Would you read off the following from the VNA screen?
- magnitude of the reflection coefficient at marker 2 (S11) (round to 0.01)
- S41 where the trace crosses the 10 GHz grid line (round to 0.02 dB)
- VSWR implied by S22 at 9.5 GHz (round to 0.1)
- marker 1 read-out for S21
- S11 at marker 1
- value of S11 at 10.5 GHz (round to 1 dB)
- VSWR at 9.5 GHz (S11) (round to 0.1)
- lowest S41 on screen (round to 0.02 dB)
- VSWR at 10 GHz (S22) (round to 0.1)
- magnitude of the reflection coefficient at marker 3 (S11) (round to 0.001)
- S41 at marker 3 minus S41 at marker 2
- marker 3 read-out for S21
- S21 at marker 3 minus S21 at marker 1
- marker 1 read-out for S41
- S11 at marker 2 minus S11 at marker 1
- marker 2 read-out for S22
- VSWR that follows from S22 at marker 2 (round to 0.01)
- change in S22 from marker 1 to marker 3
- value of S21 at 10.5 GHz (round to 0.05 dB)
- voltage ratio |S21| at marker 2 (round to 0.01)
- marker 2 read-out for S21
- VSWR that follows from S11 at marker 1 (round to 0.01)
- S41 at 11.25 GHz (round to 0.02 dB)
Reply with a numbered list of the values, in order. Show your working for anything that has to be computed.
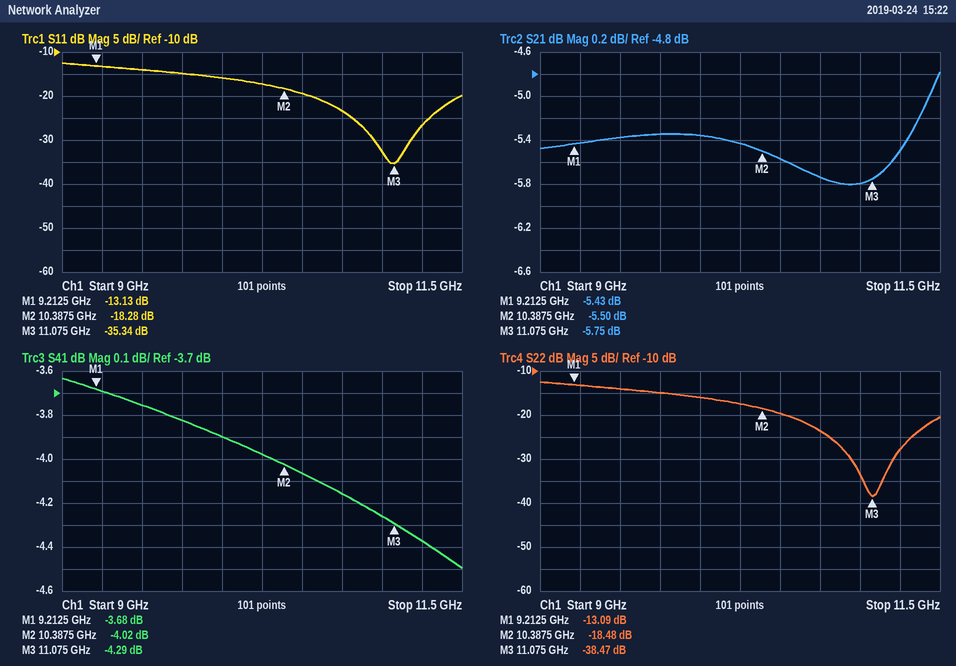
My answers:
1. 10^(-18.28/20) ≈ 0.12
2. -3.90 dB
3. |Γ| = 10^(-14/20) = 0.1995; VSWR = (1 + 0.1995)/(1 − 0.1995) ≈ 1.5
4. -5.43 dB
5. -13.13 dB
6. -19 dB
7. |Γ| = 10^(-14/20) = 0.1995; VSWR = (1 + 0.1995)/(1 − 0.1995) ≈ 1.5
8. -4.50 dB
9. |Γ| = 10^(-16/20) = 0.1585; VSWR = (1 + 0.1585)/(1 − 0.1585) ≈ 1.4
10. 10^(-35.34/20) ≈ 0.017
11. -4.29 − (-4.02) = -0.27 dB
12. -5.75 dB
13. -5.75 − (-5.43) = -0.32 dB
14. -3.68 dB
15. -18.28 − (-13.13) = -5.15 dB
16. -18.48 dB
17. (1 + 0.1191)/(1 − 0.1191) ≈ 1.27
18. -38.47 − (-13.09) = -25.38 dB
19. -5.55 dB
20. 10^(-5.5/20) ≈ 0.53
21. -5.50 dB
22. (1 + 0.2205)/(1 − 0.2205) ≈ 1.57
23. -4.38 dB
